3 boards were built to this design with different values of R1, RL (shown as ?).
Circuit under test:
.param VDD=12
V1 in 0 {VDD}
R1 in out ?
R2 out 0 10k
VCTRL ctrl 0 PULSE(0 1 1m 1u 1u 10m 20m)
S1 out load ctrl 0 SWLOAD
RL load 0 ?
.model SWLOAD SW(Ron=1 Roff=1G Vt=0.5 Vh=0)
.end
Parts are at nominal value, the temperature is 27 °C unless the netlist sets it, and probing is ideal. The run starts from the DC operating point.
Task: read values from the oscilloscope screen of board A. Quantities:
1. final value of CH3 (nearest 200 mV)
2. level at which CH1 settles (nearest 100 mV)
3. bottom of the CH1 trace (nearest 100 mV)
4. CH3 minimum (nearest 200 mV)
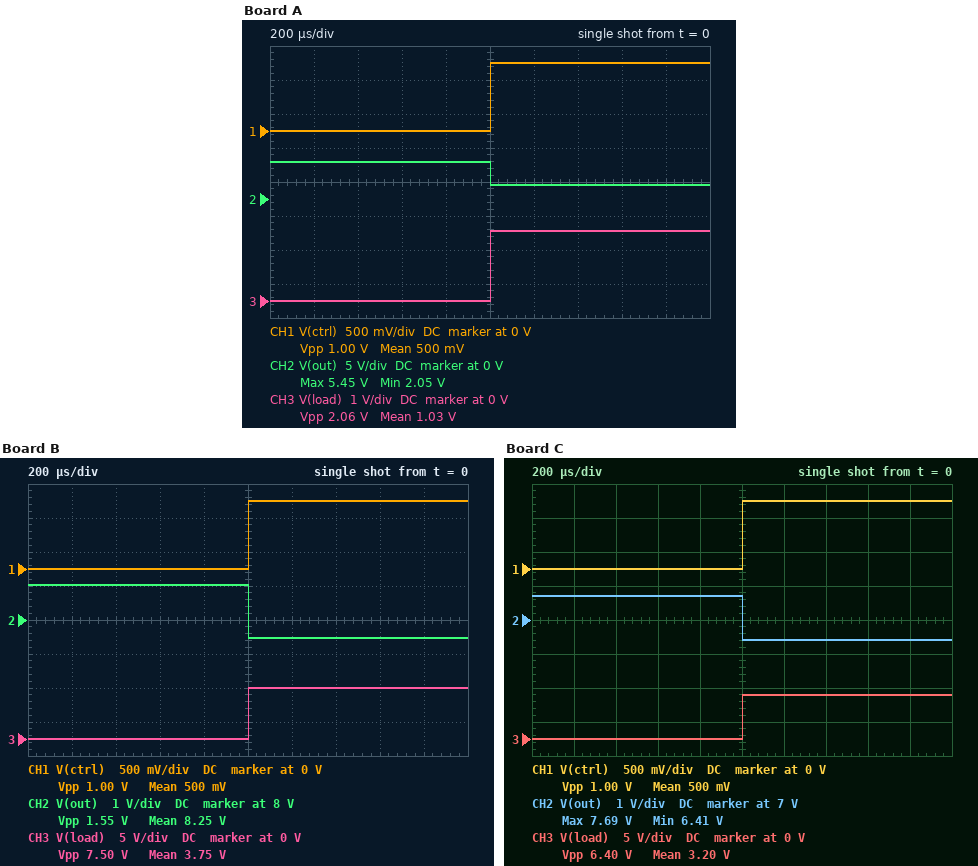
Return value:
2.0 V
1.0 V
0 V
0 V
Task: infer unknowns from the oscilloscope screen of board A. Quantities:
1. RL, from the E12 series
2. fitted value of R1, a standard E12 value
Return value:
3.3 kΩ
12 kΩ
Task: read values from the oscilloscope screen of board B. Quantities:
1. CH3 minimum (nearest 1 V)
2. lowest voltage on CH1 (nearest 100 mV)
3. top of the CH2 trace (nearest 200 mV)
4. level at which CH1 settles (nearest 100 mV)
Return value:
0 V
0 V
9.0 V
1.0 V
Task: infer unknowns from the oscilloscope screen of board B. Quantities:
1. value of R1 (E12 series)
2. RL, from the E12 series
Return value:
3.3 kΩ
12 kΩ
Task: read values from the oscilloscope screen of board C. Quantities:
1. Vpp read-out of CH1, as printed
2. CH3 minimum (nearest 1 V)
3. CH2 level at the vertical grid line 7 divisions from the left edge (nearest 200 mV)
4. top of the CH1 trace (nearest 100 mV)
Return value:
1.00 V
0 V
6.4 V
1.0 V
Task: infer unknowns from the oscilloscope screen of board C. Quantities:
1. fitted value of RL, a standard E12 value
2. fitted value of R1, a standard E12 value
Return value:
18 kΩ
5.6 kΩ
